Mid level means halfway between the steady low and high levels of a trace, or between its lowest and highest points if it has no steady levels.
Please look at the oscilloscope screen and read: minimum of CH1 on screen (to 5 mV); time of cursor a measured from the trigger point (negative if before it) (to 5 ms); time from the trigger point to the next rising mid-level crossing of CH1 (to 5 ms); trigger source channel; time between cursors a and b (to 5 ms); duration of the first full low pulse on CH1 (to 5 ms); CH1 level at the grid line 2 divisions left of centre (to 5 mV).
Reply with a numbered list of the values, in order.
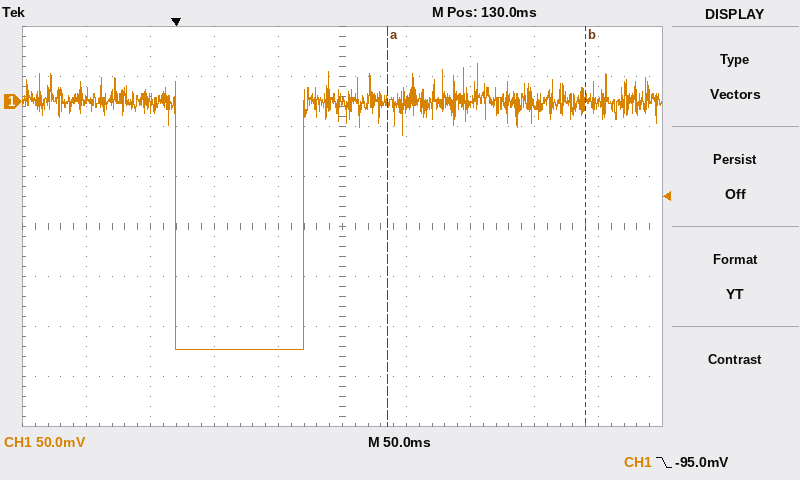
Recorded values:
1. -250 mV
2. +165 ms
3. 100 ms
4. CH1
5. 155 ms
6. 100 ms
7. -250 mV
